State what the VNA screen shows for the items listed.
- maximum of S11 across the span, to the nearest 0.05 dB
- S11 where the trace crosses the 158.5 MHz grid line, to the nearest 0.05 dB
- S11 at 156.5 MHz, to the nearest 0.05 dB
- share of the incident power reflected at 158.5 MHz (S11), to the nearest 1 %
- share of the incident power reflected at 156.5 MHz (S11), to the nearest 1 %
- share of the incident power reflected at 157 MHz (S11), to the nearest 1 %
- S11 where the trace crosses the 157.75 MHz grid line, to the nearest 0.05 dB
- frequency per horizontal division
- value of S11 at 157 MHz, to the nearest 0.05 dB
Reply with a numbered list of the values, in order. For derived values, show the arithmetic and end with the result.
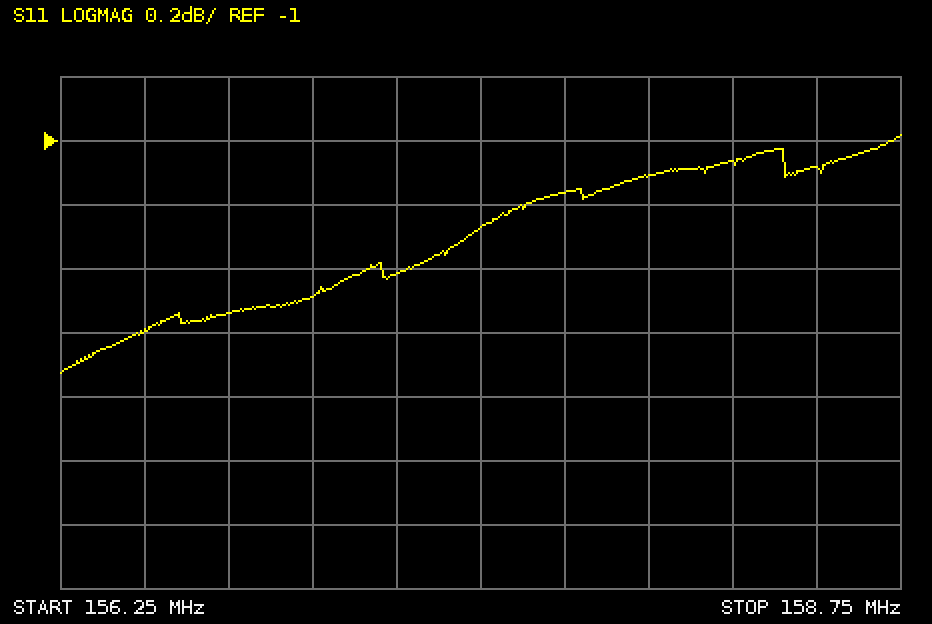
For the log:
1. -1.00 dB
2. -1.10 dB
3. -1.60 dB
4. 10^(-1.1/10) ≈ 78 %
5. 10^(-1.6/10) ≈ 69 %
6. 10^(-1.5/10) ≈ 71 %
7. -1.15 dB
8. 250 kHz
9. -1.50 dB
